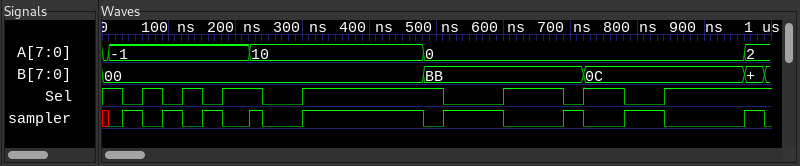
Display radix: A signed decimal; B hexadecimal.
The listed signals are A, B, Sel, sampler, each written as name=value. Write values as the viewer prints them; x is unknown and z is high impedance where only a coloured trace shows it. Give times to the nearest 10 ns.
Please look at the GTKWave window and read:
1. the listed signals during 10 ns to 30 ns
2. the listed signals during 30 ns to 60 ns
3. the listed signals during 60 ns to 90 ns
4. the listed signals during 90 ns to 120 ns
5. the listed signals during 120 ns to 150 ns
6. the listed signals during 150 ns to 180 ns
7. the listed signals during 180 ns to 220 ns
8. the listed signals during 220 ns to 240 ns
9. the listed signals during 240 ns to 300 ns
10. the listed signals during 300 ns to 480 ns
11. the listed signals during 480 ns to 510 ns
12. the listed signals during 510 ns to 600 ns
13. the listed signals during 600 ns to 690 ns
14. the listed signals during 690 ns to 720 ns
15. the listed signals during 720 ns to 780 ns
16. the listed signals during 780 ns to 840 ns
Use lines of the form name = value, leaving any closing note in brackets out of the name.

the listed signals during 10 ns to 30 ns = A=-1, B=00, Sel=1, sampler=0
the listed signals during 30 ns to 60 ns = A=-1, B=00, Sel=0, sampler=1
the listed signals during 60 ns to 90 ns = A=-1, B=00, Sel=1, sampler=0
the listed signals during 90 ns to 120 ns = A=-1, B=00, Sel=0, sampler=1
the listed signals during 120 ns to 150 ns = A=-1, B=00, Sel=1, sampler=0
the listed signals during 150 ns to 180 ns = A=-1, B=00, Sel=0, sampler=1
the listed signals during 180 ns to 220 ns = A=-1, B=00, Sel=1, sampler=0
the listed signals during 220 ns to 240 ns = A=10, B=00, Sel=1, sampler=1
the listed signals during 240 ns to 300 ns = A=10, B=00, Sel=0, sampler=0
the listed signals during 300 ns to 480 ns = A=10, B=00, Sel=1, sampler=1
the listed signals during 480 ns to 510 ns = A=0, B=BB, Sel=1, sampler=0
the listed signals during 510 ns to 600 ns = A=0, B=BB, Sel=0, sampler=1
the listed signals during 600 ns to 690 ns = A=0, B=BB, Sel=1, sampler=0
the listed signals during 690 ns to 720 ns = A=0, B=BB, Sel=0, sampler=1
the listed signals during 720 ns to 780 ns = A=0, B=0C, Sel=1, sampler=0
the listed signals during 780 ns to 840 ns = A=0, B=0C, Sel=0, sampler=1
